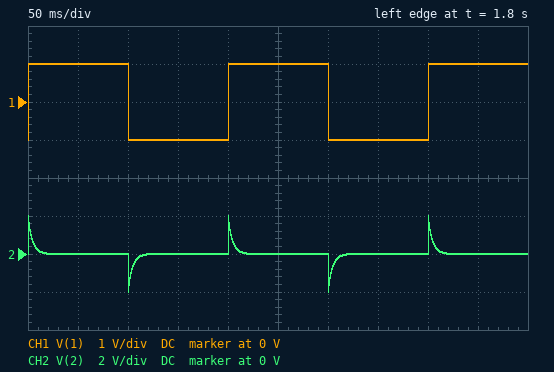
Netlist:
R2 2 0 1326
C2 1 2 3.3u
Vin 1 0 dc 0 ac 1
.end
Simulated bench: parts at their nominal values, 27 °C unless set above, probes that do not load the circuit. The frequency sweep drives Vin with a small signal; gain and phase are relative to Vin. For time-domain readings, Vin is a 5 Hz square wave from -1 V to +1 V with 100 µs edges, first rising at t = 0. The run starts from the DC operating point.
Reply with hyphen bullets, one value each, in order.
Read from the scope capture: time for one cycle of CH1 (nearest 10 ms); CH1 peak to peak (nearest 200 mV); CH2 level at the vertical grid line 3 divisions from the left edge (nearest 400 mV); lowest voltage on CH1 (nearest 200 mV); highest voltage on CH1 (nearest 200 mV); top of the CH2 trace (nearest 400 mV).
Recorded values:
- 200 ms
- 2.0 V
- 0 V
- -1.0 V
- 1.0 V
- 2.0 V
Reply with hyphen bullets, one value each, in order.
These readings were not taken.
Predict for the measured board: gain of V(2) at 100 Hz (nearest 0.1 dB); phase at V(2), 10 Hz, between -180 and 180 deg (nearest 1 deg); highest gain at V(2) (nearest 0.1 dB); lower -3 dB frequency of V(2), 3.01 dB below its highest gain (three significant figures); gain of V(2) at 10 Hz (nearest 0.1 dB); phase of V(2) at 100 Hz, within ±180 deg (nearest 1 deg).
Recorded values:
- -0.5 dB
- 75 deg
- 0 dB
- 36.4 Hz
- -11.5 dB
- 20 deg
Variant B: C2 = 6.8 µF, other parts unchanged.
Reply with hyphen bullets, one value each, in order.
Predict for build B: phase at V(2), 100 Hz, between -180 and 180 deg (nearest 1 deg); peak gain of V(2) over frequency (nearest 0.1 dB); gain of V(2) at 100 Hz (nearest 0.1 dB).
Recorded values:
- 10 deg
- 0 dB
- -0.1 dB
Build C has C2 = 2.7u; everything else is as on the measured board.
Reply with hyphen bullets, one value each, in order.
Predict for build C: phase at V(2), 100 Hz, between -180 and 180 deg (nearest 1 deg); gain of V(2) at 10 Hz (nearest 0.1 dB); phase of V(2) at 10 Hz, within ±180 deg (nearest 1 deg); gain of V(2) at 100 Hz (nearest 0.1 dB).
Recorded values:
- 24 deg
- -13.2 dB
- 77 deg
- -0.8 dB
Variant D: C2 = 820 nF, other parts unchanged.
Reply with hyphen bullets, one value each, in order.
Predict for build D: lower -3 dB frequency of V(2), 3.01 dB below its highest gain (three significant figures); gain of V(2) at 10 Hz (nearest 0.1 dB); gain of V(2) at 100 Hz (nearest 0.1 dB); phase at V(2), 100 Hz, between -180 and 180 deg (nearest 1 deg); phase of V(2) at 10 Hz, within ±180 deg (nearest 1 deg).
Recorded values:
- 146 Hz
- -23.3 dB
- -5.0 dB
- 56 deg
- 86 deg
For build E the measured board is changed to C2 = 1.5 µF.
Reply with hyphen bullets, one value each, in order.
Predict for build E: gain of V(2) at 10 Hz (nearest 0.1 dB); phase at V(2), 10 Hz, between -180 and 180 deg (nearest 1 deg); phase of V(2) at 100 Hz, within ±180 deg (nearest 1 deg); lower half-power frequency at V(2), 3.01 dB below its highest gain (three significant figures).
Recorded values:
- -18.1 dB
- 83 deg
- 39 deg
- 80.0 Hz
